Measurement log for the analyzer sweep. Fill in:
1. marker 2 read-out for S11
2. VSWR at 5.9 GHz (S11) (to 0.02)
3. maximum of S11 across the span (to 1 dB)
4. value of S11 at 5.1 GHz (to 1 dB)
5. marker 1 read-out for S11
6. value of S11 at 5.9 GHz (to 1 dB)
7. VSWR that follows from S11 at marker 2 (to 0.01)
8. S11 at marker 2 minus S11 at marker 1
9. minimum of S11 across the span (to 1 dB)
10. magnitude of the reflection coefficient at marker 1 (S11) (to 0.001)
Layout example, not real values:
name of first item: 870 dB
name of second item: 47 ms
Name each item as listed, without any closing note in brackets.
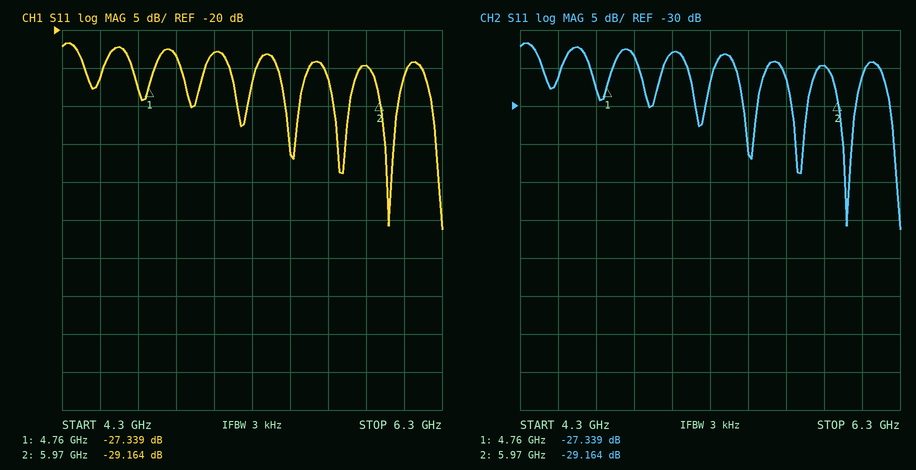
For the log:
marker 2 read-out for S11: -29.164 dB
VSWR at 5.9 GHz (S11): 1.12
maximum of S11 across the span: -22 dB
value of S11 at 5.1 GHz: -23 dB
marker 1 read-out for S11: -27.339 dB
value of S11 at 5.9 GHz: -25 dB
VSWR that follows from S11 at marker 2: 1.07
S11 at marker 2 minus S11 at marker 1: -1.825 dB
minimum of S11 across the span: -46 dB
magnitude of the reflection coefficient at marker 1 (S11): 0.043
